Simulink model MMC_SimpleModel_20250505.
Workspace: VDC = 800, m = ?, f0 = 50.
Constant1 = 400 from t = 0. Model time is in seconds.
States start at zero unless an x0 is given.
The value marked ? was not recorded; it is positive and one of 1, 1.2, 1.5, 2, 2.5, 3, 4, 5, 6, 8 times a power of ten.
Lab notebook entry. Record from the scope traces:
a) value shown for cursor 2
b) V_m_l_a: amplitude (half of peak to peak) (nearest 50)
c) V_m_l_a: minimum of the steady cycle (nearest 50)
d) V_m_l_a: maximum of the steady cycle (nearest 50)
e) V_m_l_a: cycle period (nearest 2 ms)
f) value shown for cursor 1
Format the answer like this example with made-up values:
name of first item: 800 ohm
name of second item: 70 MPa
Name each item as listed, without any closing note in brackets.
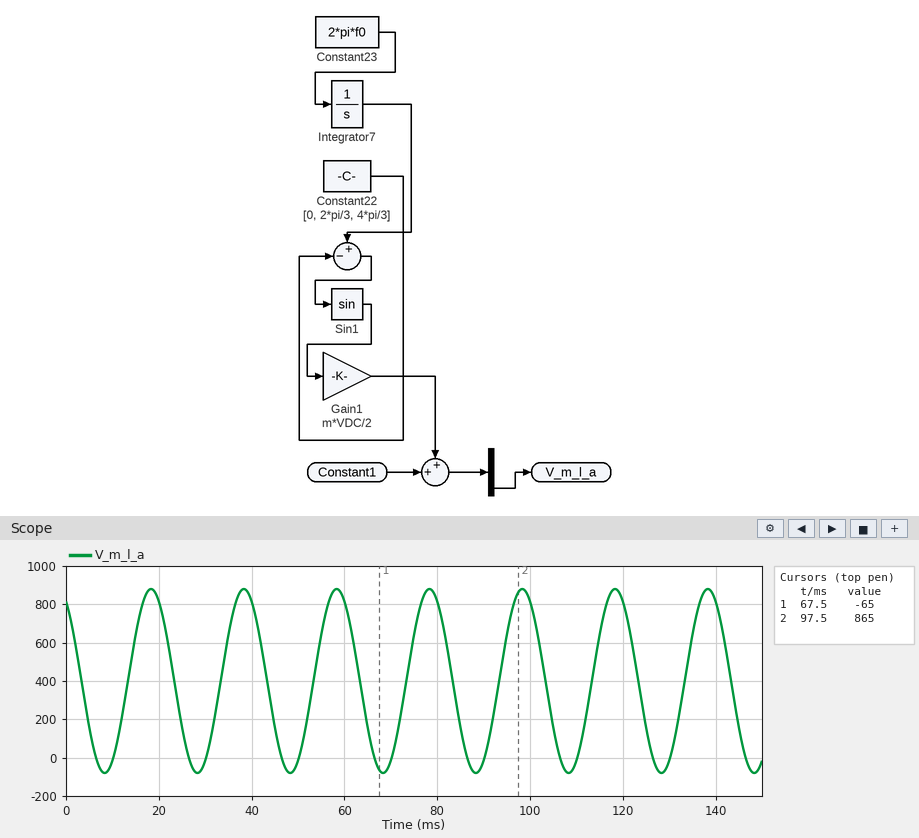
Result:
value shown for cursor 2: 865
V_m_l_a: amplitude (half of peak to peak): 500
V_m_l_a: minimum of the steady cycle: -100
V_m_l_a: maximum of the steady cycle: 900
V_m_l_a: cycle period: 20 ms
value shown for cursor 1: -65
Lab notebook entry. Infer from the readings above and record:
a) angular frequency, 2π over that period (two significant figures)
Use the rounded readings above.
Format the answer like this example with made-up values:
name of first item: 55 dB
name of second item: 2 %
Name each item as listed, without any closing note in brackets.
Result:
angular frequency, 2π over that period: 0.31 rad/ms
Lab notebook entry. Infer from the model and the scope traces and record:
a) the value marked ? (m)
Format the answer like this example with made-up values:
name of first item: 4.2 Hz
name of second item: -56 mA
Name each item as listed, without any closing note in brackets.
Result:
the value marked ?: 1.2
